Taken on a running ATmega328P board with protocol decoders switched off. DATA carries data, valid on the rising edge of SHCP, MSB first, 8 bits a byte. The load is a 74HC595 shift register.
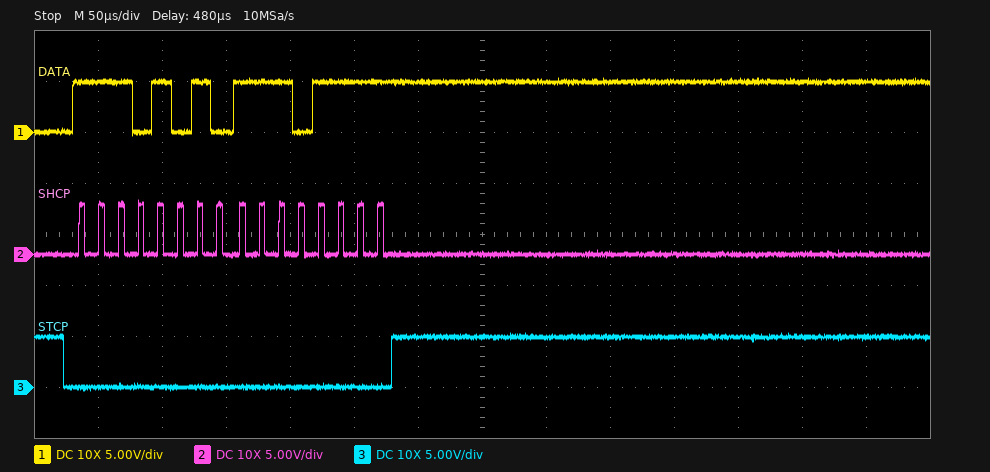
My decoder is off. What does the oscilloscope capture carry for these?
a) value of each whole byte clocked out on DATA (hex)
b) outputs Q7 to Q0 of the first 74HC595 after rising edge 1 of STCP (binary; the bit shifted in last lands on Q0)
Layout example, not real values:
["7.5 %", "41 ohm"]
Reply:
["EA EF", "11101111"]
